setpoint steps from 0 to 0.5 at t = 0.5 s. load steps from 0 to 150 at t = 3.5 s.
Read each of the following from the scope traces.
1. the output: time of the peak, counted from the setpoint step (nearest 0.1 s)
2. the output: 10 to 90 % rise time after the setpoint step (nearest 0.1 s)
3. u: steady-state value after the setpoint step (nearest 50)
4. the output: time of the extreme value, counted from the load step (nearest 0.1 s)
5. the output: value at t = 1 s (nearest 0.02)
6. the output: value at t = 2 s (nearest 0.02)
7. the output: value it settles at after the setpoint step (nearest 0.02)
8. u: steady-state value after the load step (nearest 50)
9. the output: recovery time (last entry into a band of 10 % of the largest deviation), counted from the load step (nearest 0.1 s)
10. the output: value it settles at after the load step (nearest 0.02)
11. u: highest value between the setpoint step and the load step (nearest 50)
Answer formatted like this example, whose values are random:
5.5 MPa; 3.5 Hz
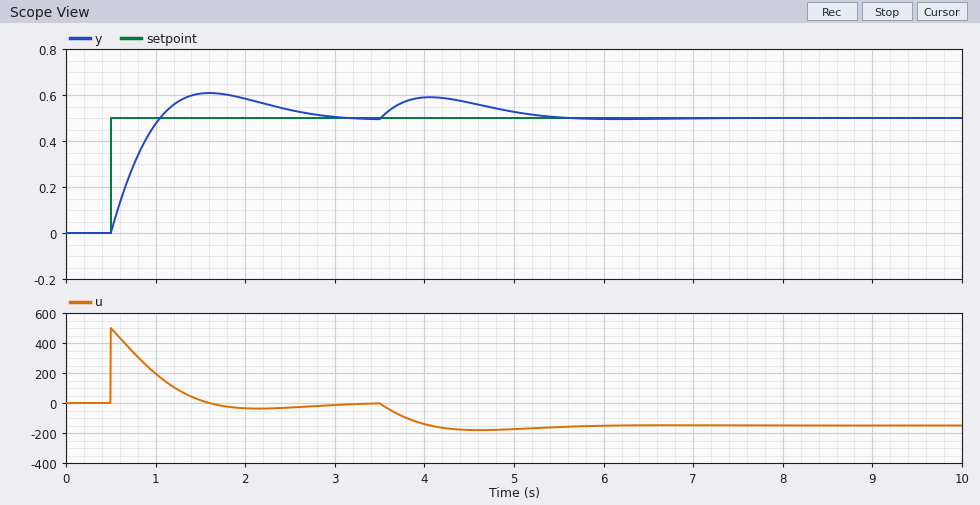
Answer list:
1.1 s; 0.4 s; 0; 0.6 s; 0.48; 0.58; 0.50; -150; 1.8 s; 0.50; 500
